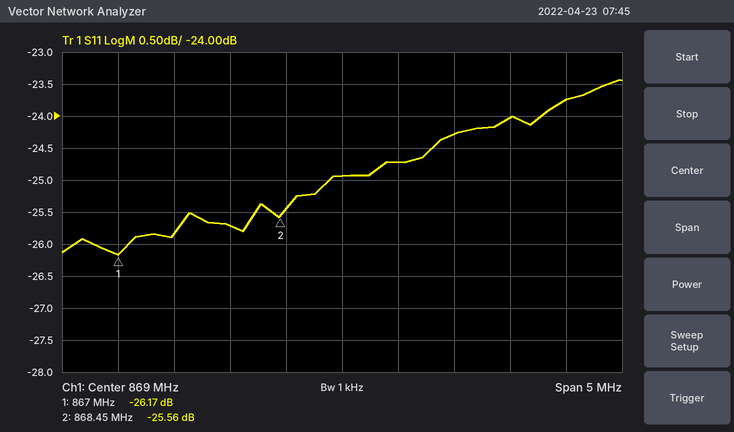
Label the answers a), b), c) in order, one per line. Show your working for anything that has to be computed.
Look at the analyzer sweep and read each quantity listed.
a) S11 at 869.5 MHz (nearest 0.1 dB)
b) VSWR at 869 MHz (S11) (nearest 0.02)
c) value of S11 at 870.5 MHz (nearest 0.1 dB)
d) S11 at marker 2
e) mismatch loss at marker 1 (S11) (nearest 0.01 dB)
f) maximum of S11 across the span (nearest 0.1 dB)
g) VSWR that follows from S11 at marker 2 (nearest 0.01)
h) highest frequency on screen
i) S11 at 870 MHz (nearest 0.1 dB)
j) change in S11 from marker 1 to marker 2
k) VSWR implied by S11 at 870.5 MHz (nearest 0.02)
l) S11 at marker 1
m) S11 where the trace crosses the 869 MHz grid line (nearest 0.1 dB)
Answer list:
a) -24.7 dB
b) |Γ| = 10^(-24.9/20) = 0.0569; VSWR = (1 + 0.0569)/(1 − 0.0569) ≈ 1.12
c) -24.0 dB
d) -25.56 dB
e) −10 log10(1 − 10^(-26.17/10)) ≈ 0.01 dB
f) -23.4 dB
g) (1 + 0.0527)/(1 − 0.0527) ≈ 1.11
h) 871.5 MHz
i) -24.3 dB
j) -25.56 − (-26.17) = 0.61 dB
k) |Γ| = 10^(-24/20) = 0.0631; VSWR = (1 + 0.0631)/(1 − 0.0631) ≈ 1.13, so 1.14 to the nearest 0.02
l) -26.17 dB
m) -24.9 dB
